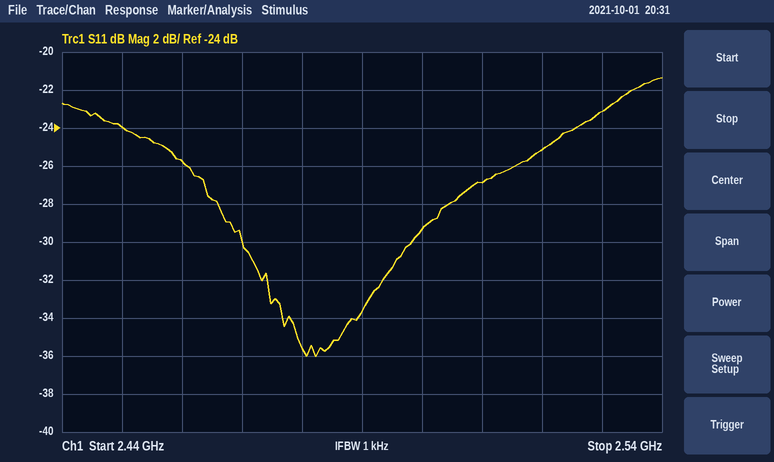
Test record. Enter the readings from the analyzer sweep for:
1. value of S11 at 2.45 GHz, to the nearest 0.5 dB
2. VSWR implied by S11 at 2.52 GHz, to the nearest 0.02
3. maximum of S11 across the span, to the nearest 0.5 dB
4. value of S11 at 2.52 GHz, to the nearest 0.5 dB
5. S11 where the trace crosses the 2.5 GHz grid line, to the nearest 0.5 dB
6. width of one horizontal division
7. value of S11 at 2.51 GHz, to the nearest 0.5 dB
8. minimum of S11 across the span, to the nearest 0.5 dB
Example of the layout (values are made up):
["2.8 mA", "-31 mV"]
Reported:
["-24.0 dB", "1.12", "-21.5 dB", "-25.0 dB", "-29.5 dB", "10 MHz", "-27.0 dB", "-36.0 dB"]
